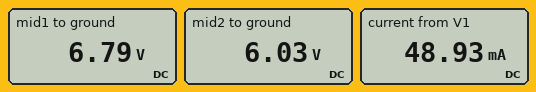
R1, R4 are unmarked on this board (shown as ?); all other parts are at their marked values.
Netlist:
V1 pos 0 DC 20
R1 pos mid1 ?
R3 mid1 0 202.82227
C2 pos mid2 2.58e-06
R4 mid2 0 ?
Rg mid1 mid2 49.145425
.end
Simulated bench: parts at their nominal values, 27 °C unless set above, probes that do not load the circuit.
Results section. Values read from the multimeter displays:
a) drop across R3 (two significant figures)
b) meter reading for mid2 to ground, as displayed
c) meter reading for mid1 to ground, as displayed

6.8 V
6.03 V
6.79 V
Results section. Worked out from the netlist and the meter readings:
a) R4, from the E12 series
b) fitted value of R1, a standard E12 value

390 Ω
270 Ω
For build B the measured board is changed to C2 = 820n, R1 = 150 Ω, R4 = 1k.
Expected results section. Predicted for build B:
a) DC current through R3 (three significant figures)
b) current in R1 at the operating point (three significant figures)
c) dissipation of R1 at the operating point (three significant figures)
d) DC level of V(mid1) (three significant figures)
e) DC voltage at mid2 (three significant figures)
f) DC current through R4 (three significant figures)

52.4 mA
62.5 mA
586 mW
10.6 V
10.1 V
10.1 mA
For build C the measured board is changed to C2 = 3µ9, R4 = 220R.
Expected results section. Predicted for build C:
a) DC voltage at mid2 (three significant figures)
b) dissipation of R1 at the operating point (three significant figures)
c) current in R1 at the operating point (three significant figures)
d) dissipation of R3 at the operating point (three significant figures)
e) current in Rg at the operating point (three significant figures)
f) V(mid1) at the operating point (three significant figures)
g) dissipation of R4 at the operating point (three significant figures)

4.90 V
726 mW
51.9 mA
177 mW
22.3 mA
6.00 V
109 mW
